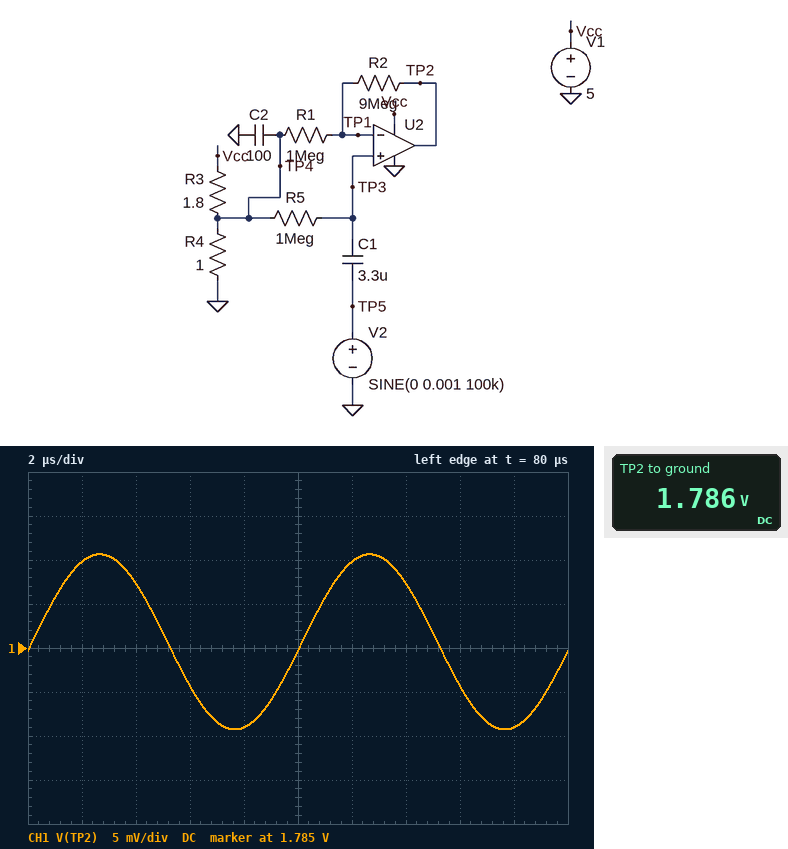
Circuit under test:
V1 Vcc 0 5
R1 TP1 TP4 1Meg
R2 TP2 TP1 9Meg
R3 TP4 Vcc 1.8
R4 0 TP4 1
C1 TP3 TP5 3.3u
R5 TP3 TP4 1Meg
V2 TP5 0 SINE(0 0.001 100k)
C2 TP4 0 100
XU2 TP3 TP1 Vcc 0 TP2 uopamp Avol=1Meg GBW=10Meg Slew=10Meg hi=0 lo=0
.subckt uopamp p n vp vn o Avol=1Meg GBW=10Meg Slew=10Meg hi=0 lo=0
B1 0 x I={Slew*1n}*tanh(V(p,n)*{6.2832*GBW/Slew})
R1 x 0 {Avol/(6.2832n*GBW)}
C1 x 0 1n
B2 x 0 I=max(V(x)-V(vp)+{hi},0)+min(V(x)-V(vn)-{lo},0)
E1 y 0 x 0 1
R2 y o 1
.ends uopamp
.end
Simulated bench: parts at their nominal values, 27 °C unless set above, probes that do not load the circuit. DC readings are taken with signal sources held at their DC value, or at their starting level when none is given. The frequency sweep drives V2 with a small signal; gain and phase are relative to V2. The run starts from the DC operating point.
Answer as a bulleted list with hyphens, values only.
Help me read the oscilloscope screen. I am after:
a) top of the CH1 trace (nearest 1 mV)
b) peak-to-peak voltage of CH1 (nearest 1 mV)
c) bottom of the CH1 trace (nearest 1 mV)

- 1.796 V
- 20 mV
- 1.776 V
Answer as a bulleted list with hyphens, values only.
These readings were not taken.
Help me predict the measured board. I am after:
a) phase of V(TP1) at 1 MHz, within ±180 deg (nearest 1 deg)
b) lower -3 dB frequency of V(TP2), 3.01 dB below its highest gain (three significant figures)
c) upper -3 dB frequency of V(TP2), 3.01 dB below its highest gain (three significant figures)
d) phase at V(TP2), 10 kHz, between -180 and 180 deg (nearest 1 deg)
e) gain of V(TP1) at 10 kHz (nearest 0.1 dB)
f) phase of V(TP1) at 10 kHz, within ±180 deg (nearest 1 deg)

- -45 deg
- 48.2 mHz
- 1.00 MHz
- -1 deg
- 0 dB
- -1 deg
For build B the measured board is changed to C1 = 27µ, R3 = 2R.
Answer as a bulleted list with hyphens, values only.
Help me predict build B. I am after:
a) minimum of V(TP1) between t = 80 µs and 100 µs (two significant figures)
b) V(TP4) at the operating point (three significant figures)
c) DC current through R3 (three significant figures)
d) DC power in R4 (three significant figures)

- 1.7 V
- 1.67 V
- 1.67 A
- 2.78 W
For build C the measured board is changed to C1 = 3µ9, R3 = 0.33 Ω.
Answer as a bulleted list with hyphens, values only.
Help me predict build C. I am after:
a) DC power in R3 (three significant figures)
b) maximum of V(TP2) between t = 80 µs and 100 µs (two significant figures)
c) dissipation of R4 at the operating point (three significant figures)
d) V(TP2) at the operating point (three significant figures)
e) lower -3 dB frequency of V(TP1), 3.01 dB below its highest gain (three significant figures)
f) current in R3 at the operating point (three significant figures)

- 4.66 W
- 3.8 V
- 14.1 W
- 3.76 V
- 40.8 mHz
- 3.76 A
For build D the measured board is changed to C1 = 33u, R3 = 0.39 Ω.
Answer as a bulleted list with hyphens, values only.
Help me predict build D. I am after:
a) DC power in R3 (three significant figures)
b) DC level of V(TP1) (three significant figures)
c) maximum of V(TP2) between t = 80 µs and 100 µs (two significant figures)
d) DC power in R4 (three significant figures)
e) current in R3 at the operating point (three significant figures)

- 5.05 W
- 3.60 V
- 3.6 V
- 12.9 W
- 3.60 A
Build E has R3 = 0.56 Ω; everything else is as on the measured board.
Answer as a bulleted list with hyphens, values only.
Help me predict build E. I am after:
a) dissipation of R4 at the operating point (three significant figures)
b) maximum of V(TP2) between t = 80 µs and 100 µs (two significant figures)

- 10.3 W
- 3.2 V
